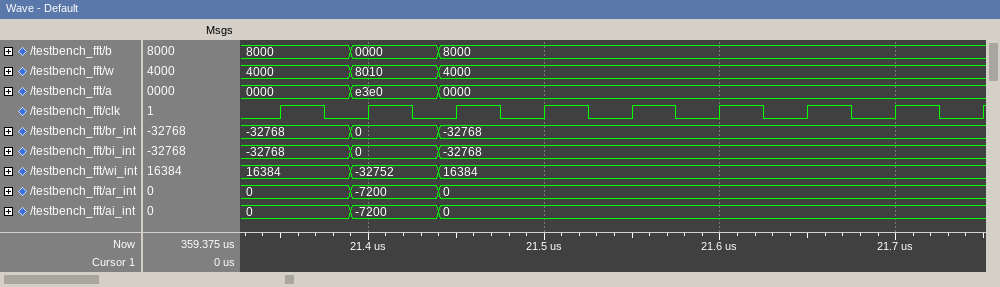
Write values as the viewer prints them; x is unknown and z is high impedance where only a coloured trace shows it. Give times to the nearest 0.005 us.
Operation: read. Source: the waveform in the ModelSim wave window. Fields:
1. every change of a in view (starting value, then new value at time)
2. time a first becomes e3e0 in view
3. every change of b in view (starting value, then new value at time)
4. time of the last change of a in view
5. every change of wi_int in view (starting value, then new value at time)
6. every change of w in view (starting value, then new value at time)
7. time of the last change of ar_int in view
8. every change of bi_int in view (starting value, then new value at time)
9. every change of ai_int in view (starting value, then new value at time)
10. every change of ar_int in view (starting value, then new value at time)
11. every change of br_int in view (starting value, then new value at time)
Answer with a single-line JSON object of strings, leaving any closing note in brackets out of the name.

{"every change of a in view": "0000, e3e0 at 21.39 us, 0000 at 21.44 us", "time a first becomes e3e0 in view": "21.39 us", "every change of b in view": "8000, 0000 at 21.39 us, 8000 at 21.44 us", "time of the last change of a in view": "21.44 us", "every change of wi_int in view": "16384, -32752 at 21.39 us, 16384 at 21.44 us", "every change of w in view": "4000, 8010 at 21.39 us, 4000 at 21.44 us", "time of the last change of ar_int in view": "21.44 us", "every change of bi_int in view": "-32768, 0 at 21.39 us, -32768 at 21.44 us", "every change of ai_int in view": "0, -7200 at 21.39 us, 0 at 21.44 us", "every change of ar_int in view": "0, -7200 at 21.39 us, 0 at 21.44 us", "every change of br_int in view": "-32768, 0 at 21.39 us, -32768 at 21.44 us"}
